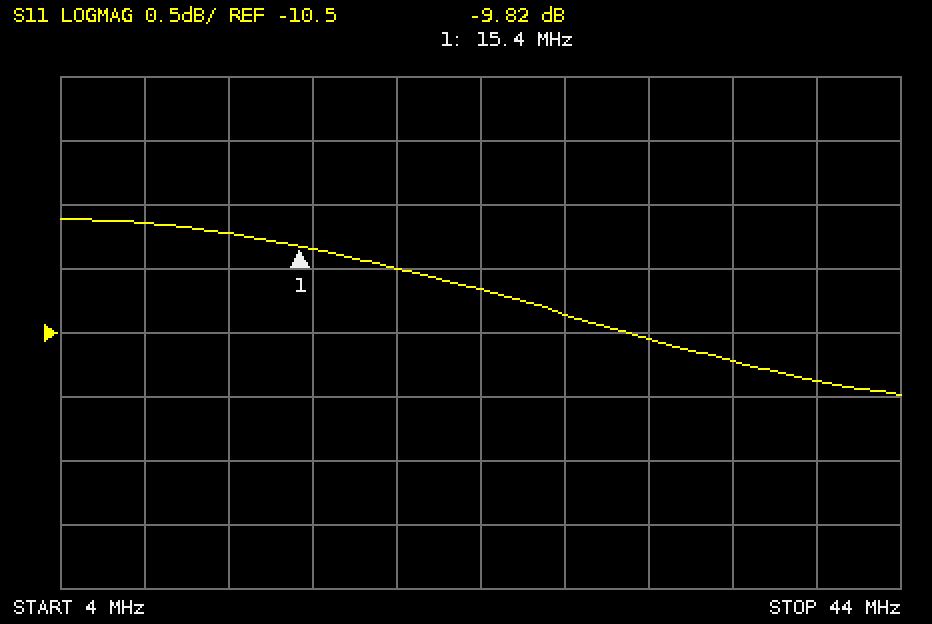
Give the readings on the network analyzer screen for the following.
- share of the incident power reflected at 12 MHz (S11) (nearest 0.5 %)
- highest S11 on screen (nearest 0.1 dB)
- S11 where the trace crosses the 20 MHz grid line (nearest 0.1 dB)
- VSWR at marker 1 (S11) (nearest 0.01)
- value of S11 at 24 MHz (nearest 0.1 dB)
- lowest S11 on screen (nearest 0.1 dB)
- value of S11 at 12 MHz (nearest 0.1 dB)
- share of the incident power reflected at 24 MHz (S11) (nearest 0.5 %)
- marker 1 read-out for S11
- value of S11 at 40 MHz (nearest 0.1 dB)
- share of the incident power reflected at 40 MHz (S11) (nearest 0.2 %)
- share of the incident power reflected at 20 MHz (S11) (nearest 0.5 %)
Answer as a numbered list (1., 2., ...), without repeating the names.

1. 10.5 %
2. -9.6 dB
3. -10.0 dB
4. 1.95
5. -10.2 dB
6. -11.0 dB
7. -9.7 dB
8. 9.5 %
9. -9.82 dB
10. -10.9 dB
11. 8.2 %
12. 10.0 %
